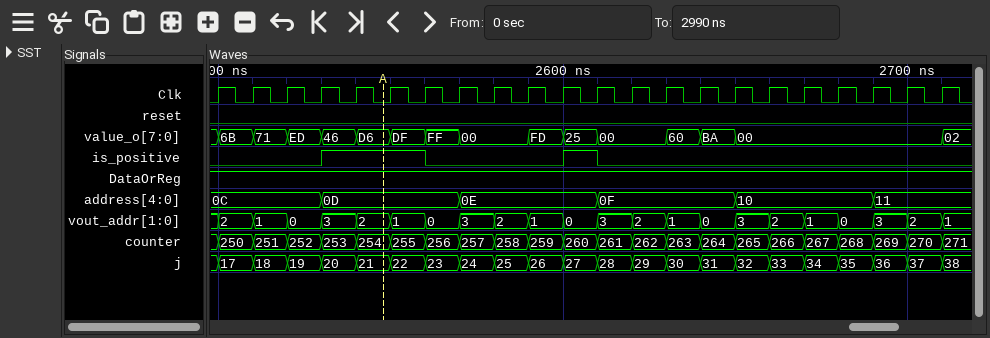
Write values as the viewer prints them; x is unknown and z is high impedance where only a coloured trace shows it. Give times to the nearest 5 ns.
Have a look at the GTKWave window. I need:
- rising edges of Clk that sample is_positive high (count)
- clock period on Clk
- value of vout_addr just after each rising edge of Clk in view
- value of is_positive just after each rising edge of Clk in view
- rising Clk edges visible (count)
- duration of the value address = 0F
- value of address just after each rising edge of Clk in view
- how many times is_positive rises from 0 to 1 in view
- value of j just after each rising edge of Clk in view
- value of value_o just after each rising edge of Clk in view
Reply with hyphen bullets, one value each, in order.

- 4
- 10 ns
- 2, 1, 0, 3, 2, 1, 0, 3, 2, 1, 0, 3, 2, 1, 0, 3, 2, 1, 0, 3, 2, 1
- 0 0 0 1 1 1 0 0 0 0 1 0 0 0 0 0 0 0 0 0 0 0
- 22
- 40 ns
- 0C, 0C, 0C, 0D, 0D, 0D, 0D, 0E, 0E, 0E, 0E, 0F, 0F, 0F, 0F, 10, 10, 10, 10, 11, 11, 11
- 2
- 17, 18, 19, 20, 21, 22, 23, 24, 25, 26, 27, 28, 29, 30, 31, 32, 33, 34, 35, 36, 37, 38
- 6B, 71, ED, 46, D6, DF, FF, 00, 00, FD, 25, 00, 00, 60, BA, 00, 00, 00, 00, 00, 00, 02
